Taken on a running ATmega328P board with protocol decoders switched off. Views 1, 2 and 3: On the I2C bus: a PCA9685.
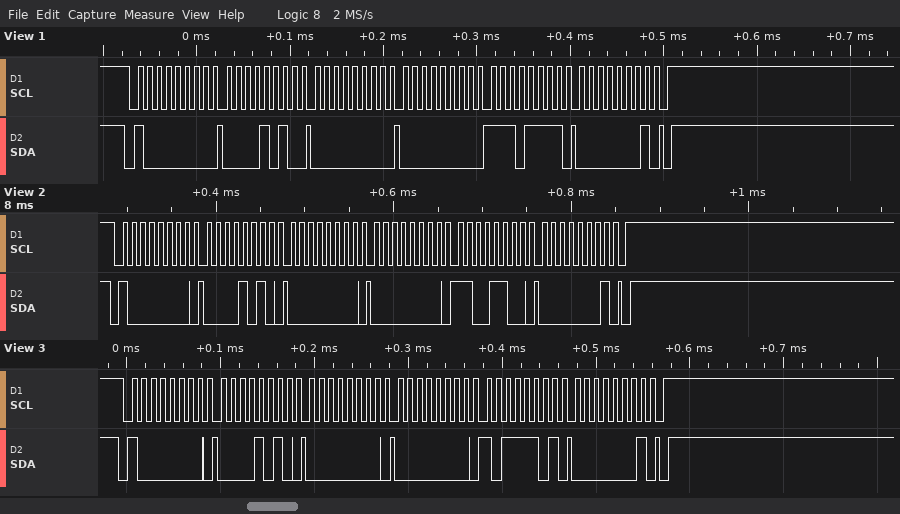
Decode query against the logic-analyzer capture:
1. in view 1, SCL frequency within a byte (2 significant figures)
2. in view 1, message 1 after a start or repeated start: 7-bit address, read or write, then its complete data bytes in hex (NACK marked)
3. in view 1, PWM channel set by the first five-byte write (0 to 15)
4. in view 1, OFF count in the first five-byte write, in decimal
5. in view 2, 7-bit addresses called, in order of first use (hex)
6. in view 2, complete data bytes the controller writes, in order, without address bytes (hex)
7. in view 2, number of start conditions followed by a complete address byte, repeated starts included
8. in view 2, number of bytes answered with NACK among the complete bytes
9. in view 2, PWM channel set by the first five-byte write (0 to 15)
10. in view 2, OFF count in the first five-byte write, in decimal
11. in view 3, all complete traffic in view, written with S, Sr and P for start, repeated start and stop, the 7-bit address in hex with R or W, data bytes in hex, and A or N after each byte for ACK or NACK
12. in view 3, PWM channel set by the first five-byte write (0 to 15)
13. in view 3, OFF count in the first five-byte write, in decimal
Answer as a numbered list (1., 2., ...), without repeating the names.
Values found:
1. 100 kHz
2. 0x40 write: 0A 00 00 EF 01
3. 1
4. 495
5. 0x40
6. 0A 00 00 CC 01
7. 1
8. 0
9. 1
10. 460
11. S 40W A 0A A 00 A 00 A BD A 01 A P
12. 1
13. 445
